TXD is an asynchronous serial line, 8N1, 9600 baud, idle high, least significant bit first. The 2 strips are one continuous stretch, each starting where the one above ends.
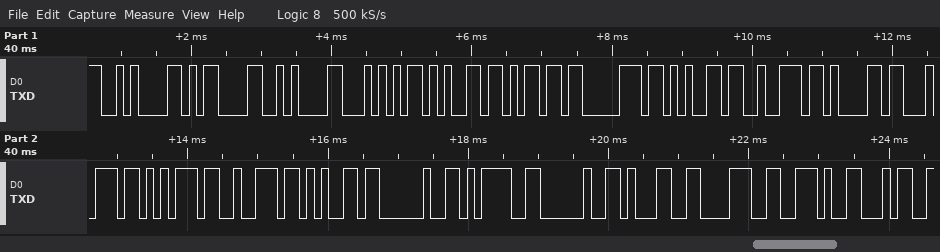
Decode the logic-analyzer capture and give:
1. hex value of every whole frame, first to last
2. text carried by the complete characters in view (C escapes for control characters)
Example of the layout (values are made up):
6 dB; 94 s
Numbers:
0A 0D 0A 54 65 6D 70 65 72 61 74 75 72 65 20 3D 20 31 38 2E 34; "\n\r\nTemperature = 18.4"
